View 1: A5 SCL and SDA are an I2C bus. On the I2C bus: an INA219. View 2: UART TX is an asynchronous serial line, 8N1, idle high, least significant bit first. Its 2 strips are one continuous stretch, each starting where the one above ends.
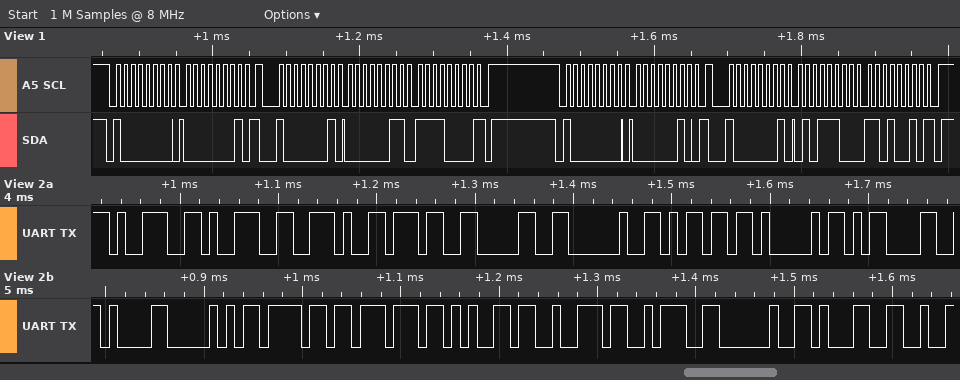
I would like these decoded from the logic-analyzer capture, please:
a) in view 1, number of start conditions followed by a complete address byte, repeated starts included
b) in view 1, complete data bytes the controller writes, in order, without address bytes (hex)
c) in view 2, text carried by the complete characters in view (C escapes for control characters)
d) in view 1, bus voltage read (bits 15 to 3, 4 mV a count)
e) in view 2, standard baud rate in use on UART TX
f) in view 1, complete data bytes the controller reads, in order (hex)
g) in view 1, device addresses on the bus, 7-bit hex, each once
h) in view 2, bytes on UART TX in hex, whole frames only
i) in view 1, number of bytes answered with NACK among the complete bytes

4
01 02
"99.70 mA\r\nPower: 1"
11.880 V
115200 baud
03 F0 5C D2
0x40
39 39 2E 37 30 20 6D 41 0D 0A 50 6F 77 65 72 3A 20 31
2
